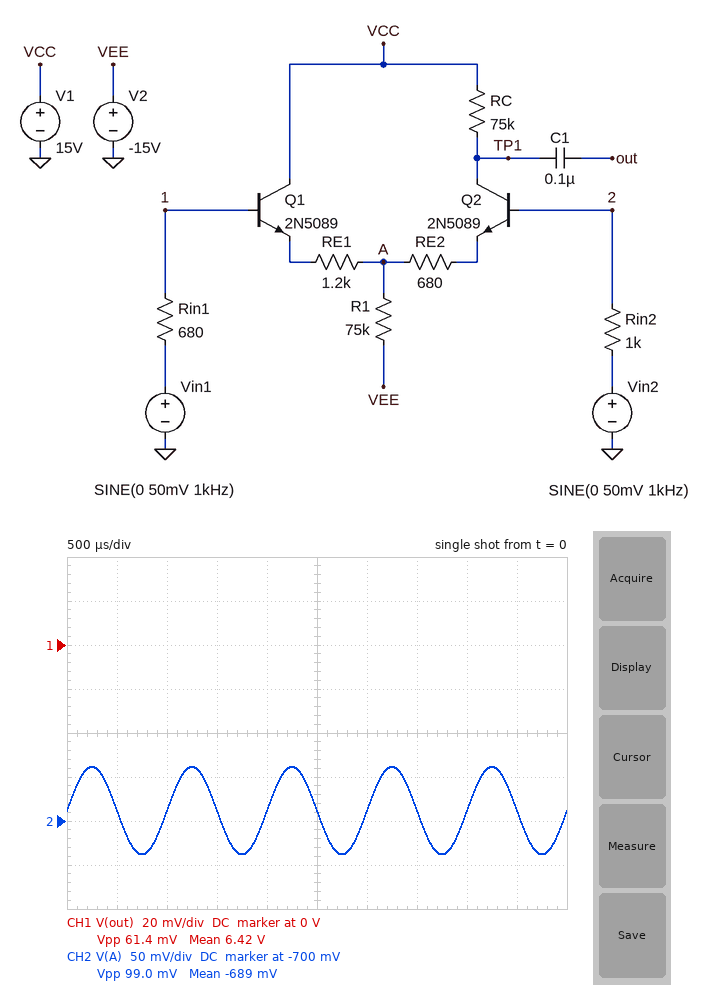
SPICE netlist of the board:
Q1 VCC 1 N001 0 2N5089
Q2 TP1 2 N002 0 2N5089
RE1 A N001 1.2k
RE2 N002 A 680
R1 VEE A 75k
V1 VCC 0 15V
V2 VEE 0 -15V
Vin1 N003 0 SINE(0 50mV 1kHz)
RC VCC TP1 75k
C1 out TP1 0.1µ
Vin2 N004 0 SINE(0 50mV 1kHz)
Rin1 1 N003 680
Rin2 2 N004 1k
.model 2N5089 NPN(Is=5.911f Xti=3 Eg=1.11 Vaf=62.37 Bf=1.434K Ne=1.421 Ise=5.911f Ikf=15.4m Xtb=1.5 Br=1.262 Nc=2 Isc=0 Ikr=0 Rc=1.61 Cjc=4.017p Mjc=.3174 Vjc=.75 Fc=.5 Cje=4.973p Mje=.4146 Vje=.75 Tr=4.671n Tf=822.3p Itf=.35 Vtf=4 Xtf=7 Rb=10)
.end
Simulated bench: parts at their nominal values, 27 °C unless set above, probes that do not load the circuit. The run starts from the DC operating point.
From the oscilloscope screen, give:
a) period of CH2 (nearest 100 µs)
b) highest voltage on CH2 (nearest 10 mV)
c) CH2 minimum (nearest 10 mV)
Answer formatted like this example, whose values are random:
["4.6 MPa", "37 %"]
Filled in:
["1.0 ms", "-640 mV", "-740 mV"]
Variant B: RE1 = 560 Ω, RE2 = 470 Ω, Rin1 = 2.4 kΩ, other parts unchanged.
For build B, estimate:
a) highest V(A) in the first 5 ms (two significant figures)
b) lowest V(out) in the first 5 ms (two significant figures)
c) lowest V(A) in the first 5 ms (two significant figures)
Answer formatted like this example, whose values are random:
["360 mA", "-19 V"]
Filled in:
["-600 mV", "7.5 V", "-700 mV"]
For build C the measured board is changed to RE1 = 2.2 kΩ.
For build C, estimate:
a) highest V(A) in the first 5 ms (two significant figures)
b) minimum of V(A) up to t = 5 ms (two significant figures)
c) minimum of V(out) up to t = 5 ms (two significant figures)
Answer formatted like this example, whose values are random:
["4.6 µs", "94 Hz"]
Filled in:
["-660 mV", "-760 mV", "4.8 V"]
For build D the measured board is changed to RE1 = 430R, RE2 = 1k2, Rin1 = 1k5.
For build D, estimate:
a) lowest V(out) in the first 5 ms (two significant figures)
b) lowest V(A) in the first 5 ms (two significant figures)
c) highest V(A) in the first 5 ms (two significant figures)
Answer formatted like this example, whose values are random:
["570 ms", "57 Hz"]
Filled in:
["10 V", "-720 mV", "-620 mV"]
